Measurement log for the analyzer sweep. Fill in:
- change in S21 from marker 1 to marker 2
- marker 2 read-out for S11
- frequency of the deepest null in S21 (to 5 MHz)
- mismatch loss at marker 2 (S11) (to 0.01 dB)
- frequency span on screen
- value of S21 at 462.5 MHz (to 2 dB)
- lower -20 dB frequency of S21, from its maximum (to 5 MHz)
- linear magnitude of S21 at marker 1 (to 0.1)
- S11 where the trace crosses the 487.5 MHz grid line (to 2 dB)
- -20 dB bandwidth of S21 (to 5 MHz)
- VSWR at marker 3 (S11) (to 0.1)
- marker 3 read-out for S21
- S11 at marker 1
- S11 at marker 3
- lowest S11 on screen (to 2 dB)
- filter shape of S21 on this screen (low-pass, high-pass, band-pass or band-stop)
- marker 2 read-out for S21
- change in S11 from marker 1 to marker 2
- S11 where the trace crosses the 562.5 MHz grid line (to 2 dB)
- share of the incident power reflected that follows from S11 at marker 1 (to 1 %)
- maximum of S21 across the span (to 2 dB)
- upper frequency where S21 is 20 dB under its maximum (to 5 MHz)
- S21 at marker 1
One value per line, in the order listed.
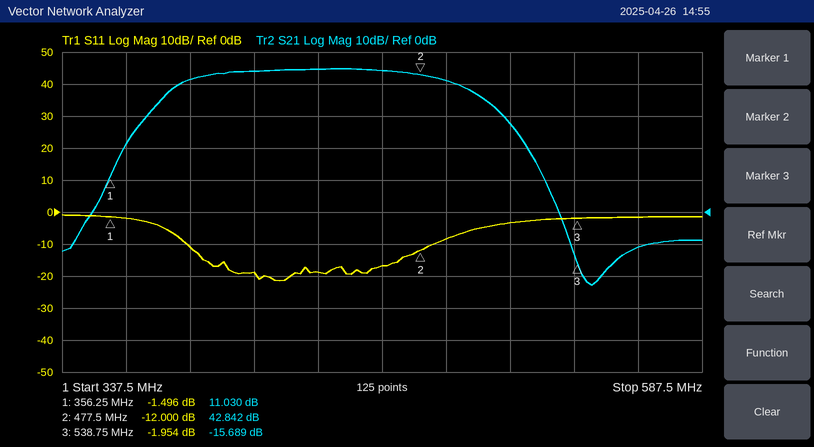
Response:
31.812 dB
-12.000 dB
545 MHz
0.28 dB
250 MHz
44 dB
365 MHz
3.6
-8 dB
150 MHz
8.9
-15.689 dB
-1.496 dB
-1.954 dB
-22 dB
band-pass
42.842 dB
-10.504 dB
-2 dB
71 %
44 dB
515 MHz
11.030 dB
